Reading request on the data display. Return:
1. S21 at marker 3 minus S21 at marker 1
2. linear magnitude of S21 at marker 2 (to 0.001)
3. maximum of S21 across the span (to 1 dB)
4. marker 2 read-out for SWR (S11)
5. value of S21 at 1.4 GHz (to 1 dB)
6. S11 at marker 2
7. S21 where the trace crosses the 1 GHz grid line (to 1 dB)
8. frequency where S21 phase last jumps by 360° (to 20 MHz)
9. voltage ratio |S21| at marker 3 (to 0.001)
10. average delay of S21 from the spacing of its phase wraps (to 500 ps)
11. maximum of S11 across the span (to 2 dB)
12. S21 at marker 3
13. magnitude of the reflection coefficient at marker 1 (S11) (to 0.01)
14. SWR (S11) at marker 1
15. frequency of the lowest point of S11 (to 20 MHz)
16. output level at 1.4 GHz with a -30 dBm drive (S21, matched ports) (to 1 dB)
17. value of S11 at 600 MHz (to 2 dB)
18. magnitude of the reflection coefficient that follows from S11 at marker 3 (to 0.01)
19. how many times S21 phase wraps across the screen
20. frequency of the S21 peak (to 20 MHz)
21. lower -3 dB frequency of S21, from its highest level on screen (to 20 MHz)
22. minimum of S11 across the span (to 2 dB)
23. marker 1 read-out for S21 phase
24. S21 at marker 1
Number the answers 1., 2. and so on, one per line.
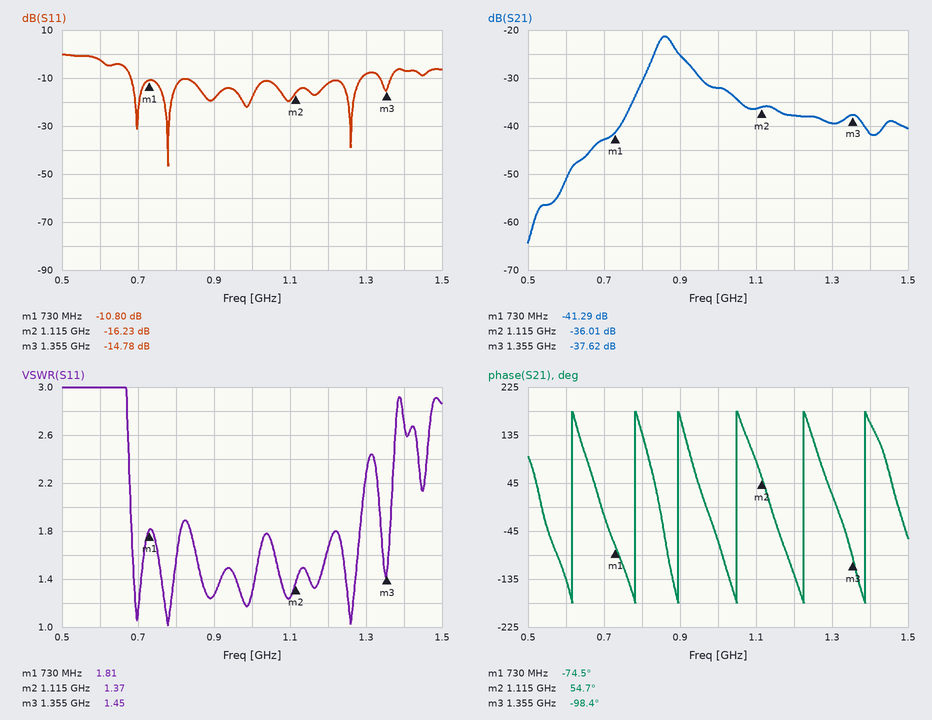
1. 3.67 dB
2. 0.016
3. -21 dB
4. 1.37
5. -42 dB
6. -16.23 dB
7. -32 dB
8. 1.38 GHz
9. 0.013
10. 6.5 ns
11. 0 dB
12. -37.62 dB
13. 0.29
14. 1.81
15. 780 MHz
16. -72 dBm
17. -2 dB
18. 0.18
19. 6
20. 860 MHz
21. 840 MHz
22. -46 dB
23. -74.5°
24. -41.29 dB
